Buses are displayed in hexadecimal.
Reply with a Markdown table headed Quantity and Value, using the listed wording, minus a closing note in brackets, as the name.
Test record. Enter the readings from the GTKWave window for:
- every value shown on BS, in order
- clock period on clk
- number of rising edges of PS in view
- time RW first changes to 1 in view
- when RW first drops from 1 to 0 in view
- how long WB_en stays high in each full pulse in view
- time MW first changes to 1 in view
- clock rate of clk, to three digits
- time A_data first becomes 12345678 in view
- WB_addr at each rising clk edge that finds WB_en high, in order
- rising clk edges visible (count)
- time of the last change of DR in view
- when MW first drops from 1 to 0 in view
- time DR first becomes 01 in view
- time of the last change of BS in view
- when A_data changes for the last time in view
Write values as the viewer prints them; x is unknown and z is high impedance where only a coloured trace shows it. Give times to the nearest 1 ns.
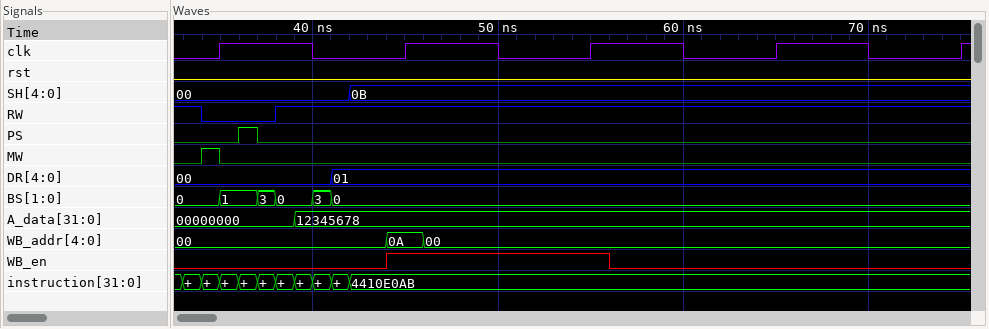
| Quantity | Value |
|---|---|
| every value shown on BS, in order | 0, 1, 3, 0, 3, 0 |
| clock period on clk | 10 ns |
| number of rising edges of PS in view | 1 |
| time RW first changes to 1 in view | 38 ns |
| when RW first drops from 1 to 0 in view | 34 ns |
| how long WB_en stays high in each full pulse in view | 12 ns |
| time MW first changes to 1 in view | 34 ns |
| clock rate of clk, to three digits | 100 MHz |
| time A_data first becomes 12345678 in view | 39 ns |
| WB_addr at each rising clk edge that finds WB_en high, in order | 0A, 00 |
| rising clk edges visible | 5 |
| time of the last change of DR in view | 41 ns |
| when MW first drops from 1 to 0 in view | 35 ns |
| time DR first becomes 01 in view | 41 ns |
| time of the last change of BS in view | 41 ns |
| when A_data changes for the last time in view | 39 ns |
